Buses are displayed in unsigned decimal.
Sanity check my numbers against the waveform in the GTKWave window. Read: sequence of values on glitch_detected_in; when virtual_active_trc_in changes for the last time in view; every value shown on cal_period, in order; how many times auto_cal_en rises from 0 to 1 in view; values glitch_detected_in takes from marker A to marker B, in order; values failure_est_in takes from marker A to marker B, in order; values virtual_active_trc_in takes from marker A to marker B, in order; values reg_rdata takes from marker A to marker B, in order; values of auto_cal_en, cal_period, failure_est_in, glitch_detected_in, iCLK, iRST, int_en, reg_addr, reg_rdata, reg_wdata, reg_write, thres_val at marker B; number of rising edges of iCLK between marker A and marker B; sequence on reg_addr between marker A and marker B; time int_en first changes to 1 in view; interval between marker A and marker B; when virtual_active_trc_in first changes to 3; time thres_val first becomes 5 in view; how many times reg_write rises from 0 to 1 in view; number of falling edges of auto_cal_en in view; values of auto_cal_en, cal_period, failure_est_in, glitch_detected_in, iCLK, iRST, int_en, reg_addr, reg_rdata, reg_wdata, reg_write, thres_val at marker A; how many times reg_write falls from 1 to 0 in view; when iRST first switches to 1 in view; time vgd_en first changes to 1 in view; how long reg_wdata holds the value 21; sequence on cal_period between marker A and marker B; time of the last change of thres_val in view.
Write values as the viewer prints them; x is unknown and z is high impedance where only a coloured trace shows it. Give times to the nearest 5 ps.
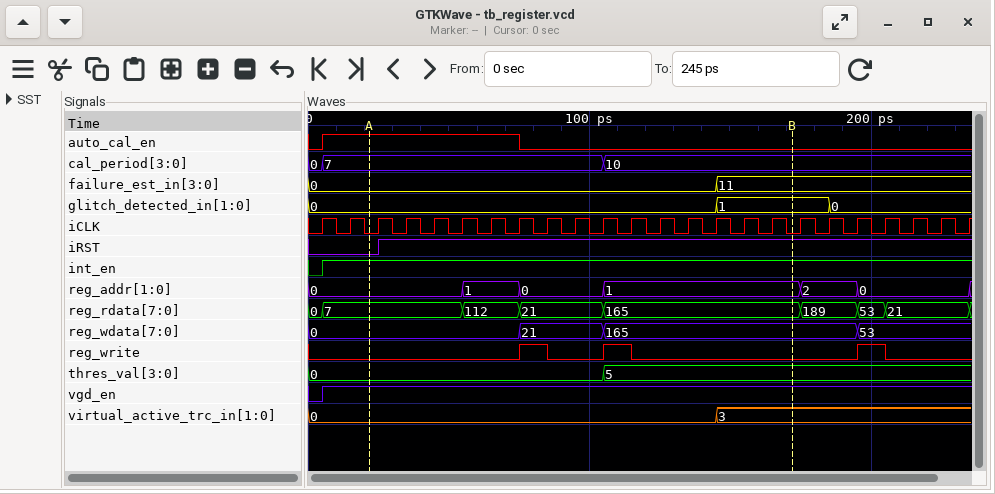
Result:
0, 1, 0
145 ps
0, 7, 10
1
0, 1
0, 11
0, 3
7, 112, 21, 165
auto_cal_en=0, cal_period=10, failure_est_in=11, glitch_detected_in=1, iCLK=0, iRST=1, int_en=1, reg_addr=1, reg_rdata=165, reg_wdata=165, reg_write=0, thres_val=5
15
0, 1, 0, 1
5 ps
150 ps
145 ps
105 ps
3
1
auto_cal_en=1, cal_period=7, failure_est_in=0, glitch_detected_in=0, iCLK=0, iRST=0, int_en=1, reg_addr=0, reg_rdata=7, reg_wdata=0, reg_write=0, thres_val=0
3
25 ps
5 ps
30 ps
7, 10
105 ps
